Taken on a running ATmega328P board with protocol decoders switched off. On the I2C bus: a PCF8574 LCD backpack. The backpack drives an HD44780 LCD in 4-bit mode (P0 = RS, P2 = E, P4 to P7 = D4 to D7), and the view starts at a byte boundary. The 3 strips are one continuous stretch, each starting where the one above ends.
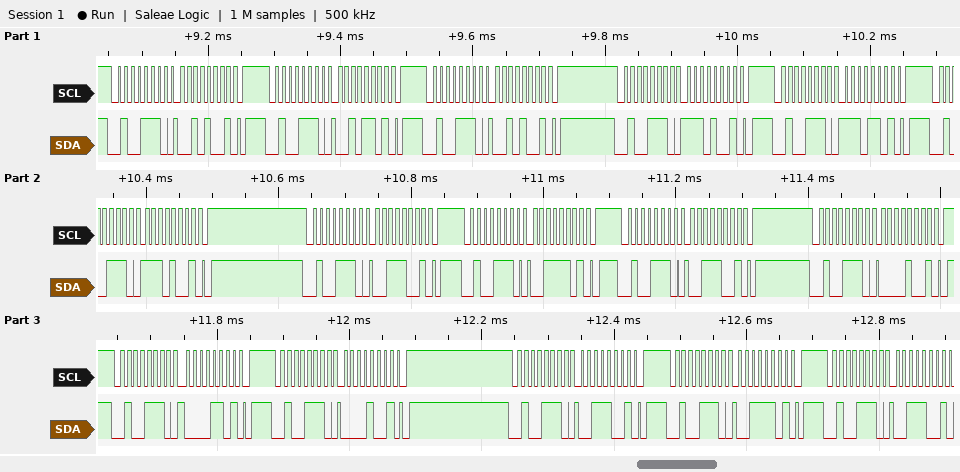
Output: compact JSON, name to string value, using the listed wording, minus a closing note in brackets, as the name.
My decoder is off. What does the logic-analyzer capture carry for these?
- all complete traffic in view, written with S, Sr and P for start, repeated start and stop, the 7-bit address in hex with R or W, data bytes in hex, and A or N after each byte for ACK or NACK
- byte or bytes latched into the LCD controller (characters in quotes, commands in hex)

{"all complete traffic in view, written with S, Sr and P for start, repeated start and stop, the 7-bit address in hex with R or W, data bytes in hex, and A or N after each byte for ACK or NACK": "S 27W A 29 A P S 27W A 2D A P S 27W A 29 A P S 27W A E9 A P S 27W A ED A P S 27W A E9 A P S 27W A 39 A P S 27W A 3D A P S 27W A 39 A P S 27W A 09 A P S 27W A 0D A P S 27W A 09 A P S 27W A 39 A P S 27W A 3D A P S 27W A 39 A", "byte or bytes latched into the LCD controller": "'.' '0'"}
